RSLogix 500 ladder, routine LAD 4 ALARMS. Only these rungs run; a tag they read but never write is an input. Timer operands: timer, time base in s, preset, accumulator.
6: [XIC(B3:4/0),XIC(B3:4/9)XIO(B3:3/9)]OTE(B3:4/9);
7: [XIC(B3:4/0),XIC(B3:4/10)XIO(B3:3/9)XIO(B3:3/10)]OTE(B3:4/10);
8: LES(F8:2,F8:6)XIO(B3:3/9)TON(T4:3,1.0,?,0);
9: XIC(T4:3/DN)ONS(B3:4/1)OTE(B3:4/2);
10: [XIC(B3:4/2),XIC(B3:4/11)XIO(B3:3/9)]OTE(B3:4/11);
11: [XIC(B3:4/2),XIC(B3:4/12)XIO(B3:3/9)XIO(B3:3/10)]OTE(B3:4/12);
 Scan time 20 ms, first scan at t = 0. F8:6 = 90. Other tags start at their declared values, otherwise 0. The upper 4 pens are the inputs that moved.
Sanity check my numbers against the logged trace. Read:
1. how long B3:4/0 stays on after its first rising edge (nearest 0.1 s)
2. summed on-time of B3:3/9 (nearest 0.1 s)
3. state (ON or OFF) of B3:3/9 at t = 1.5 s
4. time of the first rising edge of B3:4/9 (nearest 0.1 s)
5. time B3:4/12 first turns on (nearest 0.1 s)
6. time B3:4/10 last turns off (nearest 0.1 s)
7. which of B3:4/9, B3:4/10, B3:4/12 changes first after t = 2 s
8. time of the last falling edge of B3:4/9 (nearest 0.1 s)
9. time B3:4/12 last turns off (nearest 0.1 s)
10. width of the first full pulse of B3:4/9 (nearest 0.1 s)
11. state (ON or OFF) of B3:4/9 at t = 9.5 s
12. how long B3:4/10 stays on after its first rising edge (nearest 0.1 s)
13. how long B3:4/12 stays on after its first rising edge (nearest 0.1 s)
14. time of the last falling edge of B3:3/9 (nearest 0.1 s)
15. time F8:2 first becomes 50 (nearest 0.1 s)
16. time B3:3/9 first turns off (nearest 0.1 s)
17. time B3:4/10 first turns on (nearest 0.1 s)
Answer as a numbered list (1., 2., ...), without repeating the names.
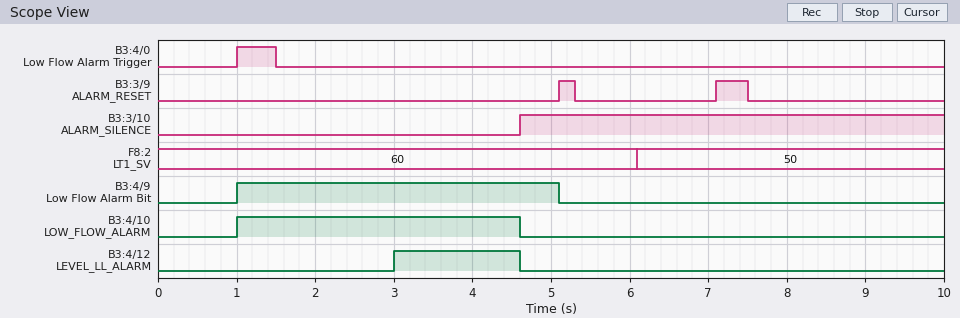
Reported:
1. 0.5 s
2. 0.6 s
3. OFF
4. 1.0 s
5. 3.0 s
6. 4.6 s
7. B3:4/12
8. 5.1 s
9. 4.6 s
10. 4.1 s
11. OFF
12. 3.6 s
13. 1.6 s
14. 7.5 s
15. 6.1 s
16. 5.3 s
17. 1.0 s
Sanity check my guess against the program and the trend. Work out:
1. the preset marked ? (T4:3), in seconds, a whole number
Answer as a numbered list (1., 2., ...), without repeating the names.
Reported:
1. 3 s
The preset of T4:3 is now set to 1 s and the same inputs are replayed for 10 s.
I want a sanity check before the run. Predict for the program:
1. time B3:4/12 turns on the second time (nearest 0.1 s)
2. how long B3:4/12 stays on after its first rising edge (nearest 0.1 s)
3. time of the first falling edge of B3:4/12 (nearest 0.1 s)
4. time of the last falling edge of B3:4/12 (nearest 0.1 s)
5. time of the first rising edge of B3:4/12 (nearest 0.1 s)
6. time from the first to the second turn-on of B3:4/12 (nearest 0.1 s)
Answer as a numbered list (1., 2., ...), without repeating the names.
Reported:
1. 6.3 s
2. 3.6 s
3. 4.6 s
4. 8.5 s
5. 1.0 s
6. 5.3 s
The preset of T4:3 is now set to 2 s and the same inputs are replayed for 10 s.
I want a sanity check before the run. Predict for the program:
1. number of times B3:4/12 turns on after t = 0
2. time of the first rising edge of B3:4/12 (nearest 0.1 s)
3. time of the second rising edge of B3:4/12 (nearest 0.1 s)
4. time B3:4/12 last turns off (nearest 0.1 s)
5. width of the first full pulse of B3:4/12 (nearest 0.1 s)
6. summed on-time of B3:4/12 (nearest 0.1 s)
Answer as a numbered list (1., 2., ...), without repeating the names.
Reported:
1. 2
2. 2.0 s
3. 9.5 s
4. 9.5 s
5. 2.6 s
6. 2.6 s
